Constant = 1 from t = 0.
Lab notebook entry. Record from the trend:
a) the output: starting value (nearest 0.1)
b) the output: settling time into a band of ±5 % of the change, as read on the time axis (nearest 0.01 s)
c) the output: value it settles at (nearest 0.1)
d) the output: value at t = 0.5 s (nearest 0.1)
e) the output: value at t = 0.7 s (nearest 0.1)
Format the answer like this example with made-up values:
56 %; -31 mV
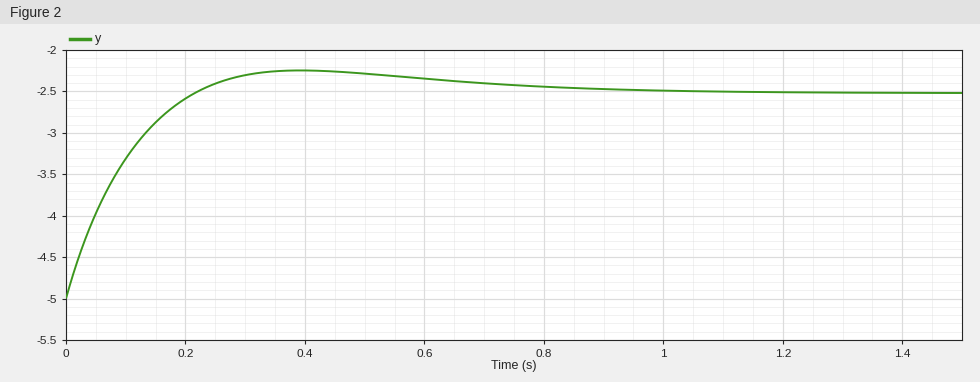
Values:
-5.0; 0.69 s; -2.5; -2.3; -2.4
